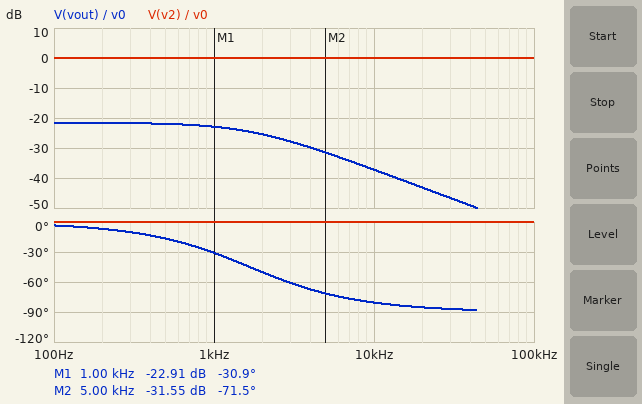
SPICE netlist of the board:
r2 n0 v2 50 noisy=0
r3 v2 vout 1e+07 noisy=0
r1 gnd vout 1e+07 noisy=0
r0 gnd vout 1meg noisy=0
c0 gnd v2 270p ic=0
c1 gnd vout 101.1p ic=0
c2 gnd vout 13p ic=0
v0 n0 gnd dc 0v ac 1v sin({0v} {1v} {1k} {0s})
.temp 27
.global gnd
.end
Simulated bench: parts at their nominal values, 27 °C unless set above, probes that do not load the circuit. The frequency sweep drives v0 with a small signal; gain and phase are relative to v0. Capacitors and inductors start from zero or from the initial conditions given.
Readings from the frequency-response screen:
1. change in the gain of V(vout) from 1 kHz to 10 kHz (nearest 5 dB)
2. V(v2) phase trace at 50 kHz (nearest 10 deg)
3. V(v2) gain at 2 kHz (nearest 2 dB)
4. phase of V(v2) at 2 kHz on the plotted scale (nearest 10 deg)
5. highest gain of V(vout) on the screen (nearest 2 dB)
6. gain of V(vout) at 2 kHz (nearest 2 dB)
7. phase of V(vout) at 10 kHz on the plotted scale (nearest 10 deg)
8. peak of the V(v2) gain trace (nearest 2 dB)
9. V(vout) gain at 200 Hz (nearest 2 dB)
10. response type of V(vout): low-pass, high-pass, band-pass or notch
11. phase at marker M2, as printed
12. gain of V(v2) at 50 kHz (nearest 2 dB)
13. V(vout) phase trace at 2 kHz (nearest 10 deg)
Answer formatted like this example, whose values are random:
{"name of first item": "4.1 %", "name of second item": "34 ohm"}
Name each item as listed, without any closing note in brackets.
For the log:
{"change in the gain of V(vout) from 1 kHz to 10 kHz": "-15 dB", "V(v2) phase trace at 50 kHz": "0 deg", "V(v2) gain at 2 kHz": "0 dB", "phase of V(v2) at 2 kHz on the plotted scale": "0 deg", "highest gain of V(vout) on the screen": "-22 dB", "gain of V(vout) at 2 kHz": "-26 dB", "phase of V(vout) at 10 kHz on the plotted scale": "-80 deg", "peak of the V(v2) gain trace": "0 dB", "V(vout) gain at 200 Hz": "-22 dB", "response type of V(vout): low-pass, high-pass, band-pass or notch": "low-pass", "phase at marker M2, as printed": "-71.5 deg", "gain of V(v2) at 50 kHz": "0 dB", "V(vout) phase trace at 2 kHz": "-50 deg"}
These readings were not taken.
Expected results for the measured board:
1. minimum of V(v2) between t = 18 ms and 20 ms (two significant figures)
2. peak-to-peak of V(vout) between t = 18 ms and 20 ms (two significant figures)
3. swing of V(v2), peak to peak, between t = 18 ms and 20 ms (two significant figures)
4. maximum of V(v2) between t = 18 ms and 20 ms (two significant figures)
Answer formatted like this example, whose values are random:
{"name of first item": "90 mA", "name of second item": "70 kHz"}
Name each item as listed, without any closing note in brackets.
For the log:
{"minimum of V(v2) between t = 18 ms and 20 ms": "-1.0 V", "peak-to-peak of V(vout) between t = 18 ms and 20 ms": "140 mV", "swing of V(v2), peak to peak, between t = 18 ms and 20 ms": "2.0 V", "maximum of V(v2) between t = 18 ms and 20 ms": "1.0 V"}
